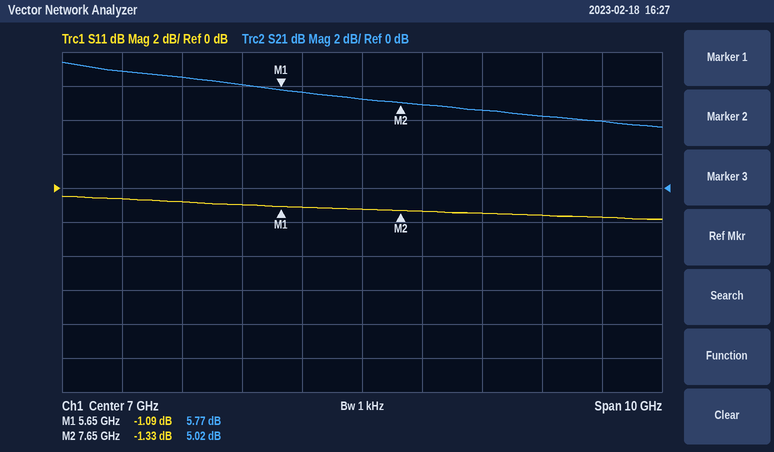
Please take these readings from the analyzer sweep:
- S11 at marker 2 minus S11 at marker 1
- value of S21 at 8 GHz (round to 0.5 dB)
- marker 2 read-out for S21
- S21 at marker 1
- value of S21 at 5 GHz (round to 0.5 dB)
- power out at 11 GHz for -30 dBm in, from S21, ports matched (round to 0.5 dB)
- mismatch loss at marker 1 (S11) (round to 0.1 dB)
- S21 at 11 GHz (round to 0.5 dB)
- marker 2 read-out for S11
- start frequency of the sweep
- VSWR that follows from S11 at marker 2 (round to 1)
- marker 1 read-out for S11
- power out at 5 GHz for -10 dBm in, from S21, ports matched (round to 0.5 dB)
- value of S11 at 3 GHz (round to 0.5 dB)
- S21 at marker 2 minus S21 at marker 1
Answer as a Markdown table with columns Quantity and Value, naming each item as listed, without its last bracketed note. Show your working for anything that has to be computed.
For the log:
| Quantity | Value |
|---|---|
| S11 at marker 2 minus S11 at marker 1 | -1.33 − (-1.09) = -0.24 dB |
| value of S21 at 8 GHz | 5.0 dB |
| marker 2 read-out for S21 | 5.02 dB |
| S21 at marker 1 | 5.77 dB |
| value of S21 at 5 GHz | 6.0 dB |
| power out at 11 GHz for -30 dBm in, from S21, ports matched | -30 dBm + (4.0 dB) = -26.0 dBm |
| mismatch loss at marker 1 (S11) | −10 log10(1 − 10^(-1.09/10)) ≈ 6.5 dB |
| S21 at 11 GHz | 4.0 dB |
| marker 2 read-out for S11 | -1.33 dB |
| start frequency of the sweep | 2 GHz |
| VSWR that follows from S11 at marker 2 | (1 + 0.8580)/(1 − 0.8580) ≈ 13 |
| marker 1 read-out for S11 | -1.09 dB |
| power out at 5 GHz for -10 dBm in, from S21, ports matched | -10 dBm + (6.0 dB) = -4.0 dBm |
| value of S11 at 3 GHz | -0.5 dB |
| S21 at marker 2 minus S21 at marker 1 | 5.02 − (5.77) = -0.75 dB |
